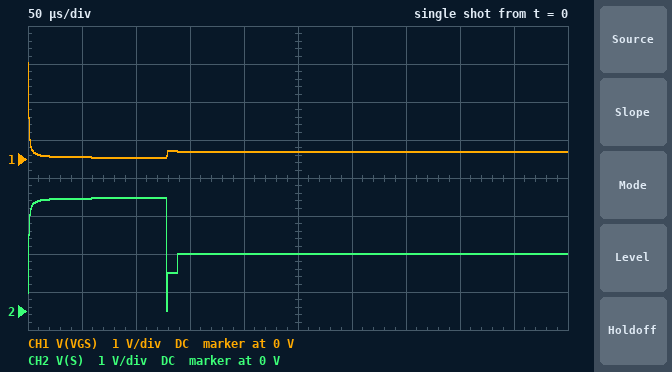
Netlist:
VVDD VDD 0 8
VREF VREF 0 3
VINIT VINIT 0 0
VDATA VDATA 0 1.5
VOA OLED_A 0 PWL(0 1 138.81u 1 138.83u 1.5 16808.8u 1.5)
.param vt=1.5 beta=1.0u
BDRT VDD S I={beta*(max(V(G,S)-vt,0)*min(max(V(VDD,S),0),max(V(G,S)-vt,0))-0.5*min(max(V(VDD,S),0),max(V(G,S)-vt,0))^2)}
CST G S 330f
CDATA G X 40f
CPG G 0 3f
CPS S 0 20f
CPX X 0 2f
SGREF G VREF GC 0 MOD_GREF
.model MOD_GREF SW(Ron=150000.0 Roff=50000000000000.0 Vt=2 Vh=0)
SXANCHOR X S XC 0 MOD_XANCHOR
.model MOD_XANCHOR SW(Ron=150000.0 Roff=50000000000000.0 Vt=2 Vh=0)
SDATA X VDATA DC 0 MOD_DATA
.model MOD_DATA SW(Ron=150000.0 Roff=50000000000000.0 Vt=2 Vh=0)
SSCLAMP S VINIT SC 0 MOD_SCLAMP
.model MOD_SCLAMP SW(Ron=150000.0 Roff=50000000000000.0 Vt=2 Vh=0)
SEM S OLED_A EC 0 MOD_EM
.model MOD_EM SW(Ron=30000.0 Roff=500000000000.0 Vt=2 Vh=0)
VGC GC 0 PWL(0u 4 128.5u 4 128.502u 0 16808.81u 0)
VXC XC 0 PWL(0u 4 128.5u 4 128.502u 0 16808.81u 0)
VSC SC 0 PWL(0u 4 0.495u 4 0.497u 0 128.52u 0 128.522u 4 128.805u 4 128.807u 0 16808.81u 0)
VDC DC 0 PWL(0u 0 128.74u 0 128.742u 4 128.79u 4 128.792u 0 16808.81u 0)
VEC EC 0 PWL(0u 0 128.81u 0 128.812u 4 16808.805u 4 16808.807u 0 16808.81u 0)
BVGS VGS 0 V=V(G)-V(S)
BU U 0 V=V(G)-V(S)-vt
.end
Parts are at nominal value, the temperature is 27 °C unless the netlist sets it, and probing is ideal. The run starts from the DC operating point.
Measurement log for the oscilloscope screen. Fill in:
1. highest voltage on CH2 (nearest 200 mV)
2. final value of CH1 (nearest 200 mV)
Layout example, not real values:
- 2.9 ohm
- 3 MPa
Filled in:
- 3.0 V
- 200 mV
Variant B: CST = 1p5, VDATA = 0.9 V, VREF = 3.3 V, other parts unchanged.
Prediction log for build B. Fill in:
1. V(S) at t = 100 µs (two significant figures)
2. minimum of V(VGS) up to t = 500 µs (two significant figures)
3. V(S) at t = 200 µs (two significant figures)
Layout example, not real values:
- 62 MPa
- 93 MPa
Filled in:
- 3.2 V
- 50 mV
- 1.5 V
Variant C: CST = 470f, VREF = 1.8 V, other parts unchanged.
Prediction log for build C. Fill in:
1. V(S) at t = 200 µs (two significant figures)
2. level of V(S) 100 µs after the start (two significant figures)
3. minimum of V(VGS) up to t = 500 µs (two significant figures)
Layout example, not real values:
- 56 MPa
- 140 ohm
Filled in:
- 1.5 V
- 1.8 V
- 34 mV
